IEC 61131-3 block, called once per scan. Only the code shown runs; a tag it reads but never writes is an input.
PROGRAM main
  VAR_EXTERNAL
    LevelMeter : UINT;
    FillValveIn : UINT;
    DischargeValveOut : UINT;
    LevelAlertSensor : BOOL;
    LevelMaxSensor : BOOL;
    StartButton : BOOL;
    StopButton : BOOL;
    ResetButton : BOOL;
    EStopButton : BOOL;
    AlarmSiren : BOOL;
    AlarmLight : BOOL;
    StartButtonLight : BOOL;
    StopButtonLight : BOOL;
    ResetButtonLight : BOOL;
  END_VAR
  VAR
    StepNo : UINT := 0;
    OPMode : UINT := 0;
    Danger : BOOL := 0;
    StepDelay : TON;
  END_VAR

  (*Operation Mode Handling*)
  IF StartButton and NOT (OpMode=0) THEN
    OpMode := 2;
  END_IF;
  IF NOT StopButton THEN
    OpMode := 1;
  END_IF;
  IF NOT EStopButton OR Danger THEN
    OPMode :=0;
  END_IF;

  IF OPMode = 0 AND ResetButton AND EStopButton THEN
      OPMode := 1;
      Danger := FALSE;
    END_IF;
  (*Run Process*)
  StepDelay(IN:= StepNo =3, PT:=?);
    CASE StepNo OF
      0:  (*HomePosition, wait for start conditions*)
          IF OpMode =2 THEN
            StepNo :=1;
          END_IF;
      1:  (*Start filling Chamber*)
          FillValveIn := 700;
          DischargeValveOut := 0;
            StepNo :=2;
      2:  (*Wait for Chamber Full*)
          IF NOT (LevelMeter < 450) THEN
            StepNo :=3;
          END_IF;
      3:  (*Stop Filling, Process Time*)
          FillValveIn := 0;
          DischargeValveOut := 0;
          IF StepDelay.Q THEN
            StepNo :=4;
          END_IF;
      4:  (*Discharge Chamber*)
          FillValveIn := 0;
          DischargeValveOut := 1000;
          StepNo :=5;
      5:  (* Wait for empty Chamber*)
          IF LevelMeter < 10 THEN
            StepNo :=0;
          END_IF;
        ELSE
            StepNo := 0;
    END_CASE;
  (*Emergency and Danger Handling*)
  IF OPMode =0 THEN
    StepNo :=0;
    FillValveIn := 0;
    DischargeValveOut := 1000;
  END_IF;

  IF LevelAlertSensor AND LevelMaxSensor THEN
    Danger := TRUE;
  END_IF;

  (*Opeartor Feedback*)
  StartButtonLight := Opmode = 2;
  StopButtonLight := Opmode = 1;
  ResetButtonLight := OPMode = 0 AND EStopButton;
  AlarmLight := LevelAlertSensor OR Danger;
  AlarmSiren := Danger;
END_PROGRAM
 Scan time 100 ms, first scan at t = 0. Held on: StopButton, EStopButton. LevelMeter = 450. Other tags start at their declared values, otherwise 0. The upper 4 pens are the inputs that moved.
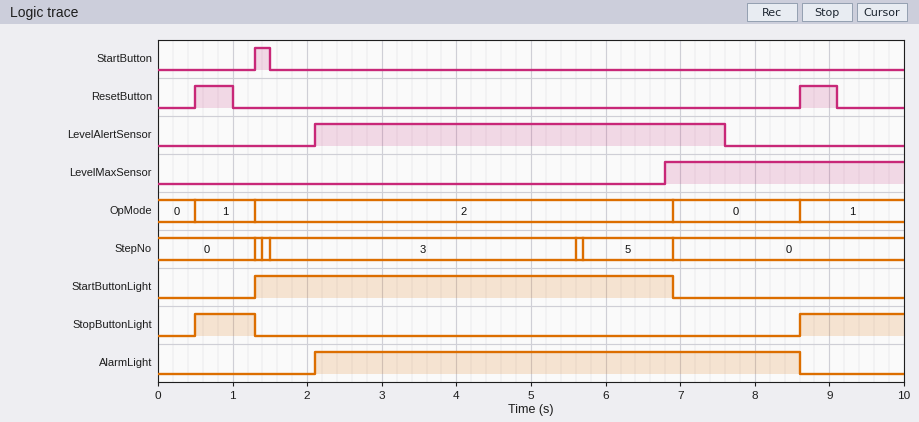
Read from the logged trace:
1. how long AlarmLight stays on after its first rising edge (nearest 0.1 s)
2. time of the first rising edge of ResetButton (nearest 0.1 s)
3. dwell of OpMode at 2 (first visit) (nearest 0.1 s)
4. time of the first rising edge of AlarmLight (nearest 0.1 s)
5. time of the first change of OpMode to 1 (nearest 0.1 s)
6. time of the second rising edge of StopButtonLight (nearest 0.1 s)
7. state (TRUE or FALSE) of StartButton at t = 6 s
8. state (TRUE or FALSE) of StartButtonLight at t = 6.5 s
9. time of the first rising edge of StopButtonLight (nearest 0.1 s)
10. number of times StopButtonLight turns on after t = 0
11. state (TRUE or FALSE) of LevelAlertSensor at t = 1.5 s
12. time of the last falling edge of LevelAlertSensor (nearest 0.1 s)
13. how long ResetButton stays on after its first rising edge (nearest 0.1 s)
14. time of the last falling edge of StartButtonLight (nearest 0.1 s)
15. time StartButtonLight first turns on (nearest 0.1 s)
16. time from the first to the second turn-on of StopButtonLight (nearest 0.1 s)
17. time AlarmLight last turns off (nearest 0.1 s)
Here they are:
6.5 s
0.5 s
5.6 s
2.1 s
0.5 s
8.6 s
FALSE
TRUE
0.5 s
2
FALSE
7.6 s
0.5 s
6.9 s
1.3 s
8.1 s
8.6 s
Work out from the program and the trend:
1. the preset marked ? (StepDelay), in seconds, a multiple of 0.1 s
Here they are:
4.0 s
